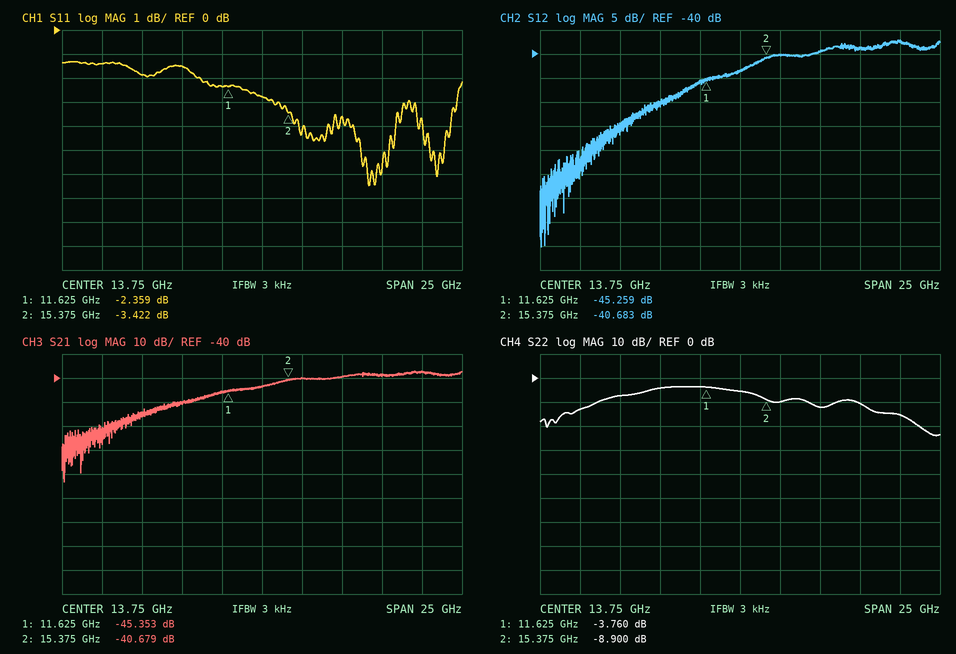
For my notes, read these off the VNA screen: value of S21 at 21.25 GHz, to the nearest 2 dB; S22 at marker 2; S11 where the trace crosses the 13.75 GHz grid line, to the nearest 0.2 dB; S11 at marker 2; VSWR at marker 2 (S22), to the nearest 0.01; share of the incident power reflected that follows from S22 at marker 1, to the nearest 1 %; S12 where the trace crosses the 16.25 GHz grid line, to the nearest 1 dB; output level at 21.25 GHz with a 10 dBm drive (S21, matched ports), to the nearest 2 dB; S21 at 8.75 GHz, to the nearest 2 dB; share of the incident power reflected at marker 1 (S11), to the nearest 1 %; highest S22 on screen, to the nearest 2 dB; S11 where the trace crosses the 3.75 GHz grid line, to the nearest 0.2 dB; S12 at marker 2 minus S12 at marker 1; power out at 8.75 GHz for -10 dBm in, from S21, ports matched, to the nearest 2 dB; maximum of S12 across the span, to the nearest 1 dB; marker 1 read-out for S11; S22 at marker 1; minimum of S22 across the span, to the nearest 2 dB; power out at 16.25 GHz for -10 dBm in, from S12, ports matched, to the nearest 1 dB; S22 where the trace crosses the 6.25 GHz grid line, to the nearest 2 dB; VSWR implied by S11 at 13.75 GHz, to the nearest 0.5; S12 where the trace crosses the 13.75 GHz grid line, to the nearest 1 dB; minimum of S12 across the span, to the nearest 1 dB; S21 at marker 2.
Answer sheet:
-38 dB
-8.900 dB
-2.8 dB
-3.422 dB
2.12
42 %
-40 dB
-28 dBm
-50 dB
58 %
-4 dB
-1.4 dB
4.576 dB
-60 dBm
-37 dB
-2.359 dB
-3.760 dB
-24 dB
-50 dBm
-8 dB
6.5
-43 dB
-80 dB
-40.679 dB
